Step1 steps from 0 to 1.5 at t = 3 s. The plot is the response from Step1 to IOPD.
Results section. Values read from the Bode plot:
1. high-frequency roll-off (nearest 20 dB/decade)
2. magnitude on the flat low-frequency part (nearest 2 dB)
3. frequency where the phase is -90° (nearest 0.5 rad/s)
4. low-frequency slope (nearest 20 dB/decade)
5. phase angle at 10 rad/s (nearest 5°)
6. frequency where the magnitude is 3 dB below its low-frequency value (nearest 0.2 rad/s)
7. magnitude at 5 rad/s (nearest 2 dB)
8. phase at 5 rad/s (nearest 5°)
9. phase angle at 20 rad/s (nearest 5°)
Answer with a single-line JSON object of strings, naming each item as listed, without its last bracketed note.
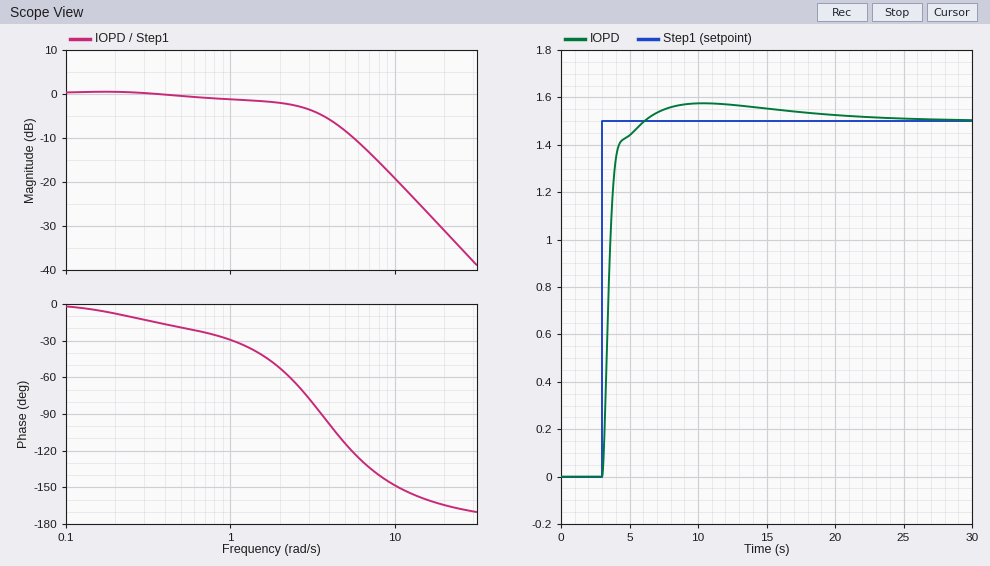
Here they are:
{"high-frequency roll-off": "-40 dB/decade", "magnitude on the flat low-frequency part": "0 dB", "frequency where the phase is -90°": "3.5 rad/s", "low-frequency slope": "0 dB/decade", "phase angle at 10 rad/s": "-150°", "frequency where the magnitude is 3 dB below its low-frequency value": "2.4 rad/s", "magnitude at 5 rad/s": "-8 dB", "phase at 5 rad/s": "-115°", "phase angle at 20 rad/s": "-165°"}
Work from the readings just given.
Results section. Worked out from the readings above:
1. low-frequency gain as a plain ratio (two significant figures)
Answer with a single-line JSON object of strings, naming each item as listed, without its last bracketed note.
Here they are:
{"low-frequency gain as a plain ratio": "1.0"}
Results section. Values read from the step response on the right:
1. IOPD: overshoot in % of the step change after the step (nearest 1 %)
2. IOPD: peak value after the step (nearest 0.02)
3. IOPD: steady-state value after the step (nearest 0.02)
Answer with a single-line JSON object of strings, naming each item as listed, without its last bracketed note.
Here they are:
{"IOPD: overshoot in % of the step change after the step": "5 %", "IOPD: peak value after the step": "1.58", "IOPD: steady-state value after the step": "1.50"}
